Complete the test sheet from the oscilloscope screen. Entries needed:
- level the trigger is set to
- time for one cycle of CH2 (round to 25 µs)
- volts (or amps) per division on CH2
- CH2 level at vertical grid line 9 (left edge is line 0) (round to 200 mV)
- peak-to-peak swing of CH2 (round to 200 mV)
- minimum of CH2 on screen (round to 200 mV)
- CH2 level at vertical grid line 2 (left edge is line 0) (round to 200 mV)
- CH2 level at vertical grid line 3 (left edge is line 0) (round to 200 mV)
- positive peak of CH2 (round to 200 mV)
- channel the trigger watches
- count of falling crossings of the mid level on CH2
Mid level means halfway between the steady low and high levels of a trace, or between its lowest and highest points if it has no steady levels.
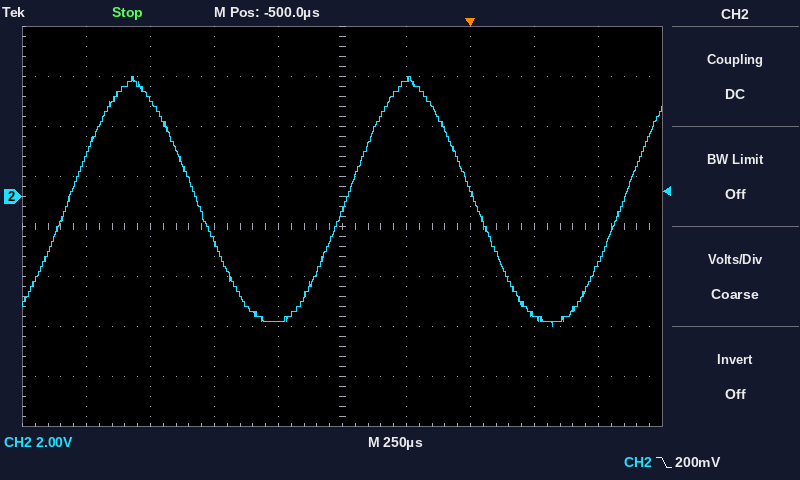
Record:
200 mV
1.075 ms
2 V
-2.6 V
10.0 V
-5.2 V
3.8 V
-1.8 V
4.8 V
CH2
2
